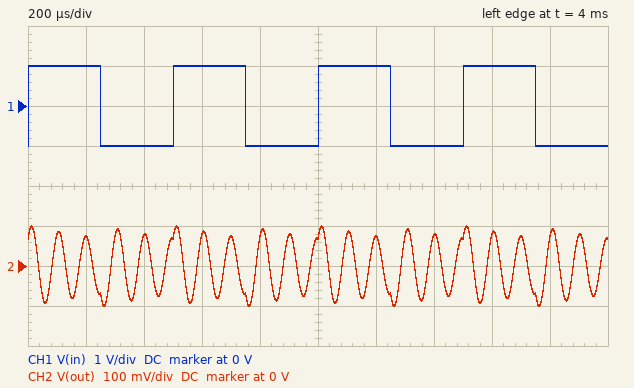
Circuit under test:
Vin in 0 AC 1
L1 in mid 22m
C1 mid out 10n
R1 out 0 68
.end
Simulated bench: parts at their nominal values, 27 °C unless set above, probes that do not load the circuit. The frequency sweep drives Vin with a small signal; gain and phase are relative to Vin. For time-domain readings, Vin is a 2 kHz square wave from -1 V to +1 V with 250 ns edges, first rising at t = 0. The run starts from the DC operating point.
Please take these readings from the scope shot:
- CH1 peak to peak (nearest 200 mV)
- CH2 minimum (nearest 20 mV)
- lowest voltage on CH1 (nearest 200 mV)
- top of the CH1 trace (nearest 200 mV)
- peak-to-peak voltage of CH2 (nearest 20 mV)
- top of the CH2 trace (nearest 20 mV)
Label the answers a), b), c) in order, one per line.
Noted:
a) 2.0 V
b) -100 mV
c) -1.0 V
d) 1.0 V
e) 200 mV
f) 100 mV
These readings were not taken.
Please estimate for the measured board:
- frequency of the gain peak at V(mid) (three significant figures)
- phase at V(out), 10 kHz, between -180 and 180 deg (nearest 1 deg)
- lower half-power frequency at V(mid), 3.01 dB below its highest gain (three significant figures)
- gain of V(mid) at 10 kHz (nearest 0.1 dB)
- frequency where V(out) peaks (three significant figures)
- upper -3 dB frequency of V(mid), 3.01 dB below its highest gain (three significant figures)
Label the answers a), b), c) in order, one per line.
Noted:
a) 10.7 kHz
b) 72 deg
c) 10.5 kHz
d) 17.2 dB
e) 10.7 kHz
f) 11.0 kHz
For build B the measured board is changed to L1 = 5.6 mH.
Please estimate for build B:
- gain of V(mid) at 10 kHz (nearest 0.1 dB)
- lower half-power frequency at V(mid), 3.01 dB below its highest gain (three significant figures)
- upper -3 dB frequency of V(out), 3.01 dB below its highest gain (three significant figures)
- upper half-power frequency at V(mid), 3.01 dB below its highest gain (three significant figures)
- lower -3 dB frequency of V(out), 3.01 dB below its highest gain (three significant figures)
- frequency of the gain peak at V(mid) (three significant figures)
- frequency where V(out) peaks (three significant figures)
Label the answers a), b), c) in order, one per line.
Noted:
a) 2.2 dB
b) 20.2 kHz
c) 22.3 kHz
d) 22.2 kHz
e) 20.3 kHz
f) 21.2 kHz
g) 21.3 kHz
